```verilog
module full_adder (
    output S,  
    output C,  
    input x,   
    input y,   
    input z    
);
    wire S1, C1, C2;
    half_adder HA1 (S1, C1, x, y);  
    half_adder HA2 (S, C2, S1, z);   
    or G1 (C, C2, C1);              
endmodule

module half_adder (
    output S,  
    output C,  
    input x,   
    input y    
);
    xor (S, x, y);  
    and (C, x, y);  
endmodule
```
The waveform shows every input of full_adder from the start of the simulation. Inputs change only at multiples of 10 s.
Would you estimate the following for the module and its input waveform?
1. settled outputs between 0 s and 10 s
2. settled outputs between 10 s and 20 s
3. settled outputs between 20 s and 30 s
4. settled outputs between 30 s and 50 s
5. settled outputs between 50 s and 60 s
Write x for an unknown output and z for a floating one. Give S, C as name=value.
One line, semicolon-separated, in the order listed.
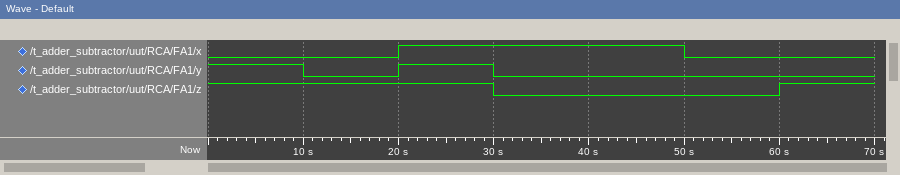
S=0, C=1; S=1, C=0; S=1, C=1; S=1, C=0; S=0, C=0
